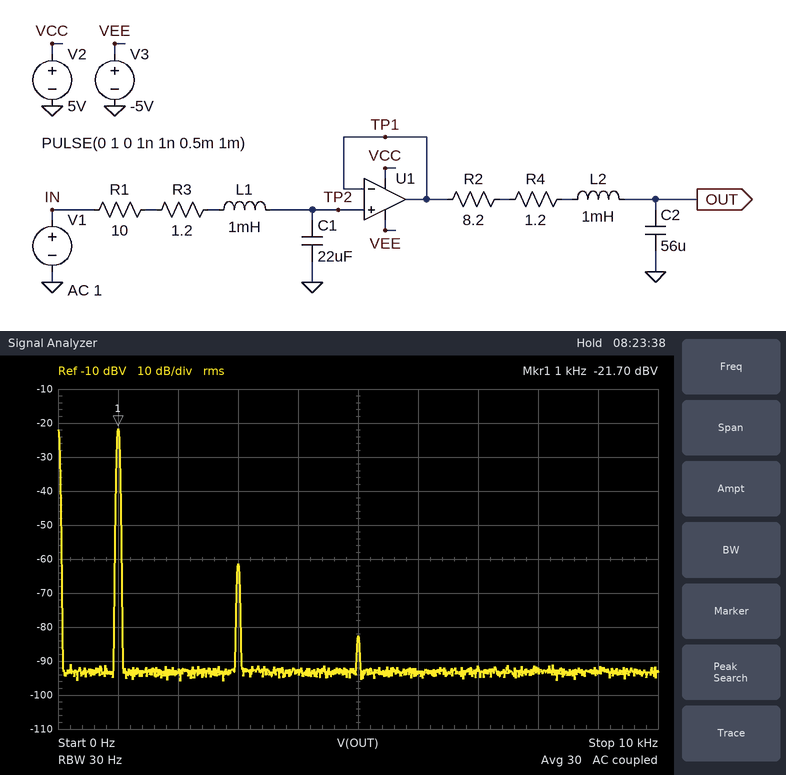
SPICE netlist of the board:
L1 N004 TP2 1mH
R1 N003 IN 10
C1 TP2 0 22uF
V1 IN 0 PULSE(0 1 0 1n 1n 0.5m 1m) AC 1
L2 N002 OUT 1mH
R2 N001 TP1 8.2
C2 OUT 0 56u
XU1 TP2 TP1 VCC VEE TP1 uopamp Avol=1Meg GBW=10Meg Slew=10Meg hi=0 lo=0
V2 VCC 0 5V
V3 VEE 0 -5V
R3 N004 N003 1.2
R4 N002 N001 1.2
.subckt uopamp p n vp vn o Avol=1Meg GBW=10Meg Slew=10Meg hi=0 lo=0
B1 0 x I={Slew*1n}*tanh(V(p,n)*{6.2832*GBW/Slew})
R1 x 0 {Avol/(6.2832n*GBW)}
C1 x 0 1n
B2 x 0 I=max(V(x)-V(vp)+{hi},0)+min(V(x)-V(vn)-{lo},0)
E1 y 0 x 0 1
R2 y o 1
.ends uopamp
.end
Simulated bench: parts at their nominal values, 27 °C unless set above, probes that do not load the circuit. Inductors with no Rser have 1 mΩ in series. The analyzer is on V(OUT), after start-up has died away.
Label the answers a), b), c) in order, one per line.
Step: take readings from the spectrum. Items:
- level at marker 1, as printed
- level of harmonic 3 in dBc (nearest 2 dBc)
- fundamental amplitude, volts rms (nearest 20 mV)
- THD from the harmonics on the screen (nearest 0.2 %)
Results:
a) -21.70 dBV
b) -40 dBc
c) 80 mV
d) 1.0 %
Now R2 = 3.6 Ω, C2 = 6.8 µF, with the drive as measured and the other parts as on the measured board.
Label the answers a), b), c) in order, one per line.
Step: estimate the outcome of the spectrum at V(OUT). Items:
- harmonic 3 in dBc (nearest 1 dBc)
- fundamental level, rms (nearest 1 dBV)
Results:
a) -30 dBc
b) -8 dBV
